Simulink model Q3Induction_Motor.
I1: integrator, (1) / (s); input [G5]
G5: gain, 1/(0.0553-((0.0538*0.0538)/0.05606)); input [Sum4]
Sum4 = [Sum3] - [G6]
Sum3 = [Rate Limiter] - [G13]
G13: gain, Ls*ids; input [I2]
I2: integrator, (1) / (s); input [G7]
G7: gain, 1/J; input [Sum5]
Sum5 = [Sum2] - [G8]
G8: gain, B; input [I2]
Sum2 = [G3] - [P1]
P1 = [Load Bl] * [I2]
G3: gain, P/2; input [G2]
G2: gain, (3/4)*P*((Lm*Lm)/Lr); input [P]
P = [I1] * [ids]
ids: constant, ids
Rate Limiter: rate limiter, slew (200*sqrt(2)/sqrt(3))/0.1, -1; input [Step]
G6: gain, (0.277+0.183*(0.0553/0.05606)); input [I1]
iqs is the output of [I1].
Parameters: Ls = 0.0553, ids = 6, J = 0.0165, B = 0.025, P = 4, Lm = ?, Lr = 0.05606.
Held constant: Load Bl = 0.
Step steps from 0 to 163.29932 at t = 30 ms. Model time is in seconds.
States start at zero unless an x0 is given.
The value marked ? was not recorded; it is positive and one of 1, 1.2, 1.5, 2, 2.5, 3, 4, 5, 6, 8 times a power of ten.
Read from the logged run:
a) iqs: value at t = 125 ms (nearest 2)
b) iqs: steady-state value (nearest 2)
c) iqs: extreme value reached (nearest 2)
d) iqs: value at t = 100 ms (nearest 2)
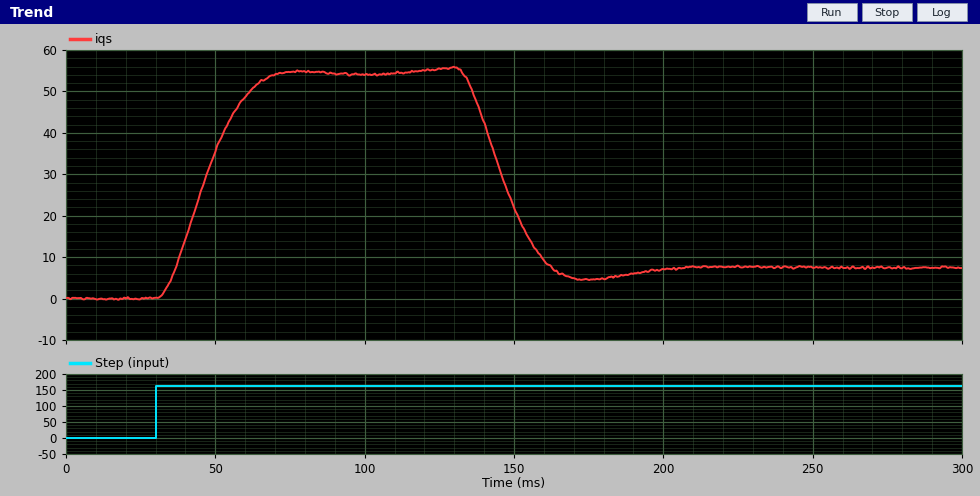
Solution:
56
8
56
54
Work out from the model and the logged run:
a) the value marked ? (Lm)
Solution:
0.05
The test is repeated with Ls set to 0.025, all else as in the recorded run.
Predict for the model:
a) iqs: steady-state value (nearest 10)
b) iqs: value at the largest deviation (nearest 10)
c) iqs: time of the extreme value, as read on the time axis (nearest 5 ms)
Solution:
20
120
130 ms
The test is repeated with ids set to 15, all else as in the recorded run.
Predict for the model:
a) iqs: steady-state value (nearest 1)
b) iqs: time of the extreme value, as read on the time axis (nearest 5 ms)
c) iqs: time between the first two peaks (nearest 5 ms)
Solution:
1
45 ms
85 ms
